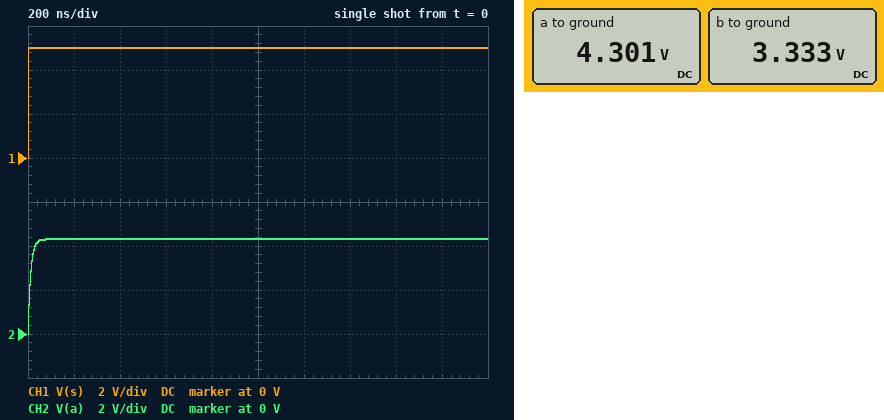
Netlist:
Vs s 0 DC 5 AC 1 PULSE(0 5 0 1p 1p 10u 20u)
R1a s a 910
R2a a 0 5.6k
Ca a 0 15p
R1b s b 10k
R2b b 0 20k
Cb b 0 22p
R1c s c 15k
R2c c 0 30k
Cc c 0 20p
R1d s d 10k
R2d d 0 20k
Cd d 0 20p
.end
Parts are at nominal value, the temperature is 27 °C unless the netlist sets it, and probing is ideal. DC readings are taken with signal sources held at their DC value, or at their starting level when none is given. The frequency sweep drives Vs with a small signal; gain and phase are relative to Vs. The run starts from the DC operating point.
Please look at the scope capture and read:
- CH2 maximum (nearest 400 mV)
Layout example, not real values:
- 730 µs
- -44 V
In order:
- 4.4 V
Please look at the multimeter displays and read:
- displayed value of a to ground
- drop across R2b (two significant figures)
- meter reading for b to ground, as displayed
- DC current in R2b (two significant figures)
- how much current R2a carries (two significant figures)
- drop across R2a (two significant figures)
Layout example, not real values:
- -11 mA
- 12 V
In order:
- 4.301 V
- 3.3 V
- 3.333 V
- 170 µA
- 770 µA
- 4.3 V
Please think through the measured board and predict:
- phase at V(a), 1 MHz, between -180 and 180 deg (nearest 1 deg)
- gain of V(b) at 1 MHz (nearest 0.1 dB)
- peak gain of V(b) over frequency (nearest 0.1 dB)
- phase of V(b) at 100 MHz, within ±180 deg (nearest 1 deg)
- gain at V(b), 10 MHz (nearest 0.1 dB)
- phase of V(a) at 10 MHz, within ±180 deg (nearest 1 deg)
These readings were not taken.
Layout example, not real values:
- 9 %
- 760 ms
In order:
- -4 deg
- -6.2 dB
- -3.5 dB
- -89 deg
- -22.9 dB
- -36 deg
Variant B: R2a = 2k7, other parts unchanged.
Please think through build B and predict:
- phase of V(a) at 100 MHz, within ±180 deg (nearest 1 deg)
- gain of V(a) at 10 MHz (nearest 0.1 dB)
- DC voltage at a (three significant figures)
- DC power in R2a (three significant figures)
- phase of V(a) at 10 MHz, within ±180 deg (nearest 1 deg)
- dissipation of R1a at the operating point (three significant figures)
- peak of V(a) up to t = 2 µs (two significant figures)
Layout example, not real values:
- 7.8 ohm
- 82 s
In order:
- -81 deg
- -4.0 dB
- 3.74 V
- 5.18 mW
- -33 deg
- 1.75 mW
- 3.7 V
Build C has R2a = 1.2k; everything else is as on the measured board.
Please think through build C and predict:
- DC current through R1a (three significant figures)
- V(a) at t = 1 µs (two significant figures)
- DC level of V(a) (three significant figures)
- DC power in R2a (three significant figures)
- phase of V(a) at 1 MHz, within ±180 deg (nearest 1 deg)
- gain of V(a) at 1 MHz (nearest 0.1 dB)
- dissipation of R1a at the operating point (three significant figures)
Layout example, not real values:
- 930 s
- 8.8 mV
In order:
- 2.37 mA
- 2.8 V
- 2.84 V
- 6.74 mW
- -3 deg
- -4.9 dB
- 5.11 mW
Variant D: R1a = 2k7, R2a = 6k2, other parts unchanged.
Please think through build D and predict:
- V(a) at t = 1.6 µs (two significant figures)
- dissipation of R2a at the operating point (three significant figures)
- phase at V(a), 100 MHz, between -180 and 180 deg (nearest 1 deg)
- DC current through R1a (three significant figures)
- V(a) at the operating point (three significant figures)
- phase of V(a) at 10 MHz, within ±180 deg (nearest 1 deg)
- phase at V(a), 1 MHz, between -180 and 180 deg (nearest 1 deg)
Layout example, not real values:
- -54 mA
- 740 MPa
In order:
- 3.5 V
- 1.96 mW
- -87 deg
- 562 µA
- 3.48 V
- -61 deg
- -10 deg
